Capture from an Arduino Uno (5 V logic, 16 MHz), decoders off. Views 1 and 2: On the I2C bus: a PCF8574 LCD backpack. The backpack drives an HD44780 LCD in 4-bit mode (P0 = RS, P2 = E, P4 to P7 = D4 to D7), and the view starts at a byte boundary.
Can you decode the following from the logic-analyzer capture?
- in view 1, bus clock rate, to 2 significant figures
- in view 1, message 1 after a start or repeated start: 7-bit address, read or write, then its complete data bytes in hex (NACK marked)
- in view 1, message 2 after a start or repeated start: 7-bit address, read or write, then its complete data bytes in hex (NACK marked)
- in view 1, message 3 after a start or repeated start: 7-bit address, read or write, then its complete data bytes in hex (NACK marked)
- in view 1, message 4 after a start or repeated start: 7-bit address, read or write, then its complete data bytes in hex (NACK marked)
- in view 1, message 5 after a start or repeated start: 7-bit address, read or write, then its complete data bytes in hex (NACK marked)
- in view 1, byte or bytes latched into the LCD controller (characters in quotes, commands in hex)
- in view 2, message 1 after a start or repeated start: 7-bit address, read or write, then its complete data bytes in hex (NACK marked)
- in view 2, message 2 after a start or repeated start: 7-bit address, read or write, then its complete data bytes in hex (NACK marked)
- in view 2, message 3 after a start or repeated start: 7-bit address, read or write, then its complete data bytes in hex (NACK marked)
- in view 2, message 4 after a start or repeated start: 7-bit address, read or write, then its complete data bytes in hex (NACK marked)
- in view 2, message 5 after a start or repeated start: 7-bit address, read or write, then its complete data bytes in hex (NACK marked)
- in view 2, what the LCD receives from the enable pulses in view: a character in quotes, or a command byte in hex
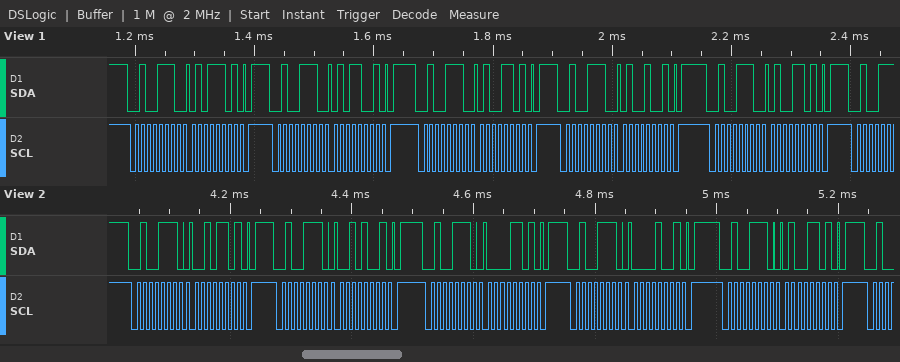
100 kHz
0x27 write: 5D
0x27 write: 59
0x27 write: 4D
0x27 write: 49
0x27 write: 4D
'T'
0x27 write: 2D
0x27 write: 29
0x27 write: 0D
0x27 write: 09
0x27 write: 4D
' '
